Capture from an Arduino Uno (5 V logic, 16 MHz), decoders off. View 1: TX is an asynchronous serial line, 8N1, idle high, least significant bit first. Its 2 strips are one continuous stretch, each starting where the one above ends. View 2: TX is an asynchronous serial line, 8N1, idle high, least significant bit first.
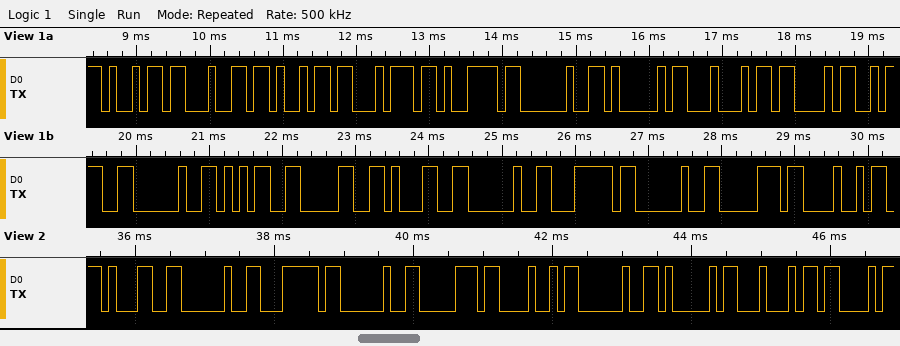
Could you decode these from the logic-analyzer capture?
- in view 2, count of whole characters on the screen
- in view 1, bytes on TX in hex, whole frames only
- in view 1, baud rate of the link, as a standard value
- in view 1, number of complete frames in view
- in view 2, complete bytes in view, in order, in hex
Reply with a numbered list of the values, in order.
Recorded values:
1. 10
2. 69 64 69 74 79 20 41 44 43 3A 20 35 30 31 20 7C 20 70 48
3. 9600 baud
4. 19
5. 31 20 7C 20 70 48 20 41 44 43
